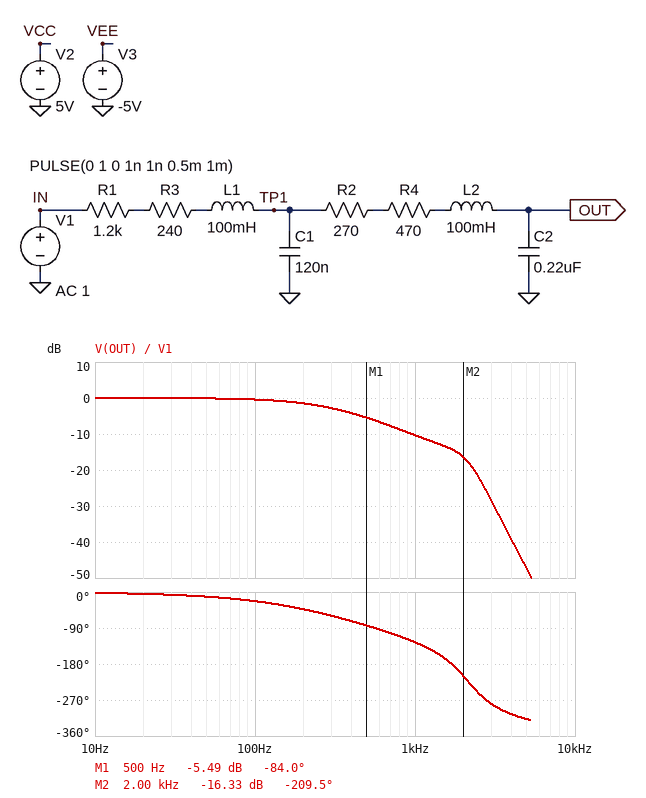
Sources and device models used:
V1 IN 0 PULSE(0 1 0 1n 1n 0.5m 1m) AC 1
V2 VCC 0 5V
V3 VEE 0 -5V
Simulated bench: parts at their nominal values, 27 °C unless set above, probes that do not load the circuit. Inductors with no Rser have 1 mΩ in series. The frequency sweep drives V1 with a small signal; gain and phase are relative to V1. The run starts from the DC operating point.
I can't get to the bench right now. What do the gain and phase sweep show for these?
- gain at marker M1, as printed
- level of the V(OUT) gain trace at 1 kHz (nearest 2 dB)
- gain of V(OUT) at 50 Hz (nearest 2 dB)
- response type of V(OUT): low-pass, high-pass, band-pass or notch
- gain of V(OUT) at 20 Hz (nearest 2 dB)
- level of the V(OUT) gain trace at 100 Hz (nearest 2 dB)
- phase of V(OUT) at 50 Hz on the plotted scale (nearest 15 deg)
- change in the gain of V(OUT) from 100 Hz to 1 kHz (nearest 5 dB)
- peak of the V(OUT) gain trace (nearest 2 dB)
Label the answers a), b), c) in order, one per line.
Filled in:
a) -5.49 dB
b) -10 dB
c) 0 dB
d) low-pass
e) 0 dB
f) 0 dB
g) -15 deg
h) -10 dB
i) 0 dB
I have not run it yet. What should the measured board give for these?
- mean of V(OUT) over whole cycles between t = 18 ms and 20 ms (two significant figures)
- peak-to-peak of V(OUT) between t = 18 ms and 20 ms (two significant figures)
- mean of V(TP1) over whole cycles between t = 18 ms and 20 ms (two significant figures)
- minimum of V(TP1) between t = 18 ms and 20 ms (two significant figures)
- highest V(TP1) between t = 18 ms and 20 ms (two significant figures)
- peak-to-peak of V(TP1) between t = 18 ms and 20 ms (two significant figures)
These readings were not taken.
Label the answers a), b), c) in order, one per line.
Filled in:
a) 500 mV
b) 390 mV
c) 500 mV
d) 300 mV
e) 700 mV
f) 390 mV
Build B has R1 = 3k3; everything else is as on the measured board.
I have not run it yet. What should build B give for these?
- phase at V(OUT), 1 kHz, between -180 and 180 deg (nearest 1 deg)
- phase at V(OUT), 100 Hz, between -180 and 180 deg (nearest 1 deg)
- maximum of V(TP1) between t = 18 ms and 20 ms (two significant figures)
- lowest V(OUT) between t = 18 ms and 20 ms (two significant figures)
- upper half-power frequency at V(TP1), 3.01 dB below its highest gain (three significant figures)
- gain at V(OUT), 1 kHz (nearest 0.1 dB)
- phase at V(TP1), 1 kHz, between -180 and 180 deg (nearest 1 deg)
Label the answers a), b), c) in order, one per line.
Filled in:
a) -121 deg
b) -42 deg
c) 600 mV
d) 400 mV
e) 124 Hz
f) -16.6 dB
g) -39 deg
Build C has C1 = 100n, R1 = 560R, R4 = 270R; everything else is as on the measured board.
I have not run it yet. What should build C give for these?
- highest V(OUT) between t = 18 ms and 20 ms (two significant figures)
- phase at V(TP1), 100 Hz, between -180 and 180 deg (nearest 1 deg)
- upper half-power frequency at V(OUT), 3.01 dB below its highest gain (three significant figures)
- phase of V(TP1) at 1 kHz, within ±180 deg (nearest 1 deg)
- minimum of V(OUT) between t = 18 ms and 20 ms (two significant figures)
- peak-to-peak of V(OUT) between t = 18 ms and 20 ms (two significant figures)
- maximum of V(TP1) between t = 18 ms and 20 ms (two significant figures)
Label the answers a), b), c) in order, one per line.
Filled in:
a) 820 mV
b) -9 deg
c) 706 Hz
d) -46 deg
e) 180 mV
f) 640 mV
g) 770 mV
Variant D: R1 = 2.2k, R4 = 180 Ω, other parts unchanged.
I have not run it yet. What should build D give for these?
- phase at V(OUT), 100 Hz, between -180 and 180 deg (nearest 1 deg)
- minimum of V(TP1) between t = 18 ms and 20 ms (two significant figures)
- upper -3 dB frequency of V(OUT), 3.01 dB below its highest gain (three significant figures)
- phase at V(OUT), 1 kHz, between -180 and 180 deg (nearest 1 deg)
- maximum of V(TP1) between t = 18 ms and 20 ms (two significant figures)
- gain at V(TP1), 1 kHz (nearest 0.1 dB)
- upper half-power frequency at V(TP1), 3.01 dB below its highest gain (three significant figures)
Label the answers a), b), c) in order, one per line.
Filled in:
a) -31 deg
b) 390 mV
c) 193 Hz
d) -116 deg
e) 610 mV
f) -16.8 dB
g) 184 Hz
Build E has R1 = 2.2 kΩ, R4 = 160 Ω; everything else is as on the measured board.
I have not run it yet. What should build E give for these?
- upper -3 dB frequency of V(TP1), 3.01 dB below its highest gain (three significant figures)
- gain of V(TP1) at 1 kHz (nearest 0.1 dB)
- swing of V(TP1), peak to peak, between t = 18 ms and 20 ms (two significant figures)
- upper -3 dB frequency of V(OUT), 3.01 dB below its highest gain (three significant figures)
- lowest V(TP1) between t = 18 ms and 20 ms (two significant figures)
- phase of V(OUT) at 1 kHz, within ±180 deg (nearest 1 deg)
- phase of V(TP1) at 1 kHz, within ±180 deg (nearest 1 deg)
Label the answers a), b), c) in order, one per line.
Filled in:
a) 184 Hz
b) -17.1 dB
c) 220 mV
d) 193 Hz
e) 390 mV
f) -116 deg
g) -38 deg
